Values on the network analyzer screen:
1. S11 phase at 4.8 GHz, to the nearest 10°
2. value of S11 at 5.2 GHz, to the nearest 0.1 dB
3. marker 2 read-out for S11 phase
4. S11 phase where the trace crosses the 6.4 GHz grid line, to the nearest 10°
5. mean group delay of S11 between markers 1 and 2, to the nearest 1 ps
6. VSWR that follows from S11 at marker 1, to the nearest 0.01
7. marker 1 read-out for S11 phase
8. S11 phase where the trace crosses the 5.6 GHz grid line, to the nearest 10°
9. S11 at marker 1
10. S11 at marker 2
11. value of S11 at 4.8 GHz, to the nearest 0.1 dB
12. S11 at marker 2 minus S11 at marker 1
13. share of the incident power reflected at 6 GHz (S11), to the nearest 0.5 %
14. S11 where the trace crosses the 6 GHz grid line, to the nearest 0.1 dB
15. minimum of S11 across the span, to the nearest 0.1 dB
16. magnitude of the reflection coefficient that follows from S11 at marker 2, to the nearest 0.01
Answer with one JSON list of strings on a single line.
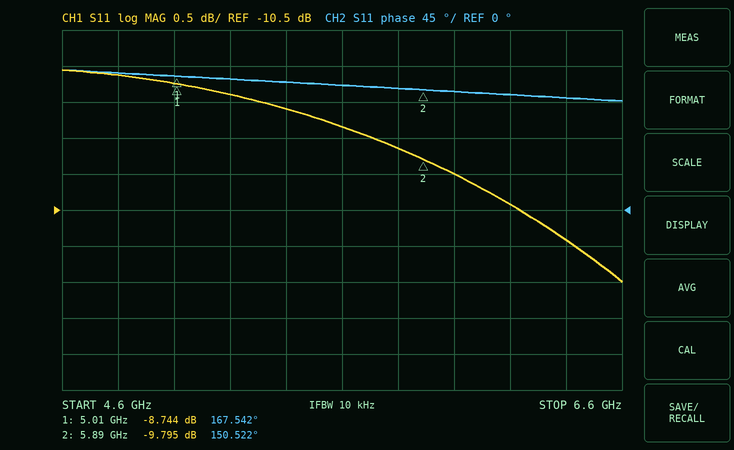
["170°", "-8.9 dB", "150.522°", "140°", "54 ps", "2.15", "167.542°", "160°", "-8.744 dB", "-9.795 dB", "-8.6 dB", "-1.051 dB", "10.0 %", "-10.0 dB", "-11.5 dB", "0.32"]
